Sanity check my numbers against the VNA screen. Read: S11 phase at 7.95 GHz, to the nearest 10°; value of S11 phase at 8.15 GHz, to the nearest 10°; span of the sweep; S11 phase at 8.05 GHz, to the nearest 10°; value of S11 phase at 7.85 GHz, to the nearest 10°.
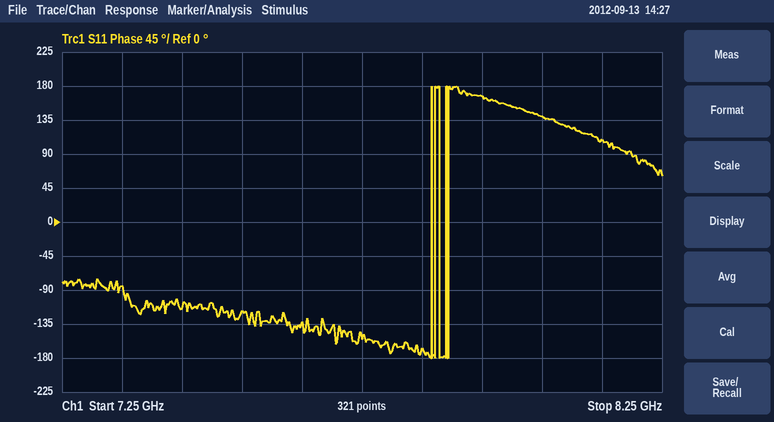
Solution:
170°
110°
1 GHz
140°
-170°
